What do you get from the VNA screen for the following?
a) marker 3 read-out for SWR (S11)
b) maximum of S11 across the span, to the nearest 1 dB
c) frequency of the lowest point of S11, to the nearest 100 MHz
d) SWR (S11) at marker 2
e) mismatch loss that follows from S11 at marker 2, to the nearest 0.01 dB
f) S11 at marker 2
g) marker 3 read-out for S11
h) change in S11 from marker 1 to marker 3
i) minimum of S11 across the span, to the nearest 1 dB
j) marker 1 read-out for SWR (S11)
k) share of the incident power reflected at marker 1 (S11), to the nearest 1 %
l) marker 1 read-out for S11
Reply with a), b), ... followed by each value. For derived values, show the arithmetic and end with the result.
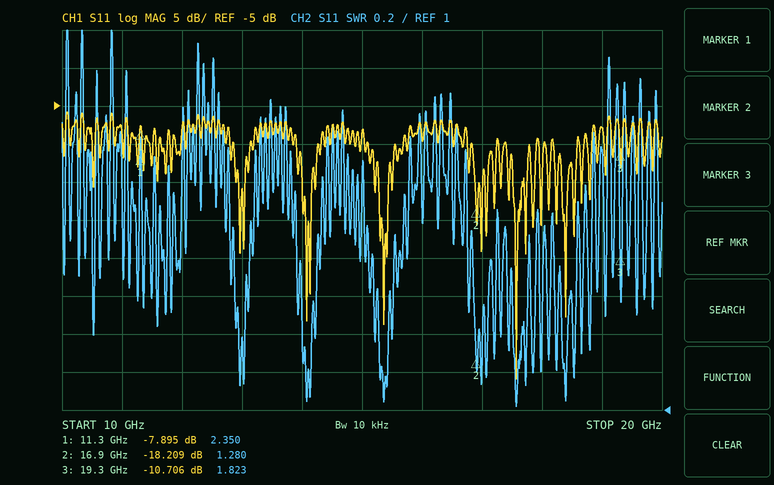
a) 1.823
b) -6 dB
c) 17.6 GHz
d) 1.280
e) −10 log10(1 − 10^(-18.209/10)) ≈ 0.07 dB
f) -18.209 dB
g) -10.706 dB
h) -10.706 − (-7.895) = -2.811 dB
i) -41 dB
j) 2.350
k) 10^(-7.895/10) ≈ 16 %
l) -7.895 dB
